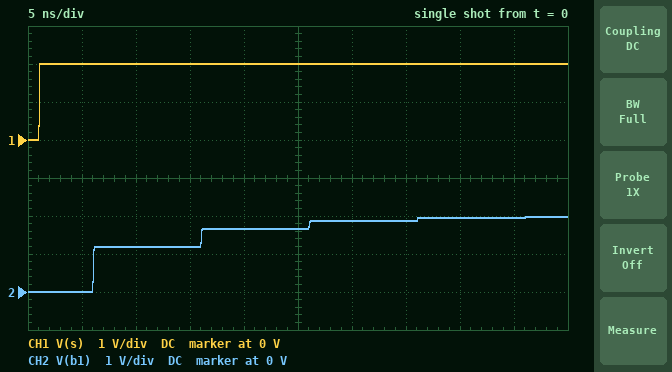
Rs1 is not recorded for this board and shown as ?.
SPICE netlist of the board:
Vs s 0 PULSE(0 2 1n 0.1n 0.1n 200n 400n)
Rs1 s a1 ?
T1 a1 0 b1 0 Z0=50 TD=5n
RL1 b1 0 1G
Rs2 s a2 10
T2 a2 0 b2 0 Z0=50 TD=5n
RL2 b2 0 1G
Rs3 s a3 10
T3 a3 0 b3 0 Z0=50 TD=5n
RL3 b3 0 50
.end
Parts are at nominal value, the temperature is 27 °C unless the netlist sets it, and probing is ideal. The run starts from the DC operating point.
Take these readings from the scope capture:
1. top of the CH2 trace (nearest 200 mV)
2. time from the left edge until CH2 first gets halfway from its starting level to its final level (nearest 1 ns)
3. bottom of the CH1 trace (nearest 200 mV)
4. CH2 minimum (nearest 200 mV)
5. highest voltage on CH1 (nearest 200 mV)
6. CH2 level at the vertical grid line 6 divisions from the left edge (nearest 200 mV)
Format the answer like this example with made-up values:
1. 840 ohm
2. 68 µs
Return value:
1. 2.0 V
2. 6 ns
3. 0 V
4. 0 V
5. 2.0 V
6. 1.8 V
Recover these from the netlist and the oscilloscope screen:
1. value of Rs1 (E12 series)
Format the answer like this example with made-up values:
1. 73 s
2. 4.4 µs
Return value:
1. 120 Ω
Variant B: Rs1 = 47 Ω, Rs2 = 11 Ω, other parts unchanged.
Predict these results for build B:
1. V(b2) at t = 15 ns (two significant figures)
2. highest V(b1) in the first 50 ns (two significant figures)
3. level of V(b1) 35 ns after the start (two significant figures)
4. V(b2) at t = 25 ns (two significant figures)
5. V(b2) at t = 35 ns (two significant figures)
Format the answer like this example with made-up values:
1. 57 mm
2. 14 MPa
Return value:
1. 3.3 V
2. 2.1 V
3. 2.0 V
4. 1.2 V
5. 2.5 V
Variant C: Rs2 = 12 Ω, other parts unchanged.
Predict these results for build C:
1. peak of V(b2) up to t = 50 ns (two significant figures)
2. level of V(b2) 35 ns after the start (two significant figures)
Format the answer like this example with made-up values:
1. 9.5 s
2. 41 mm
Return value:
1. 3.2 V
2. 2.5 V
